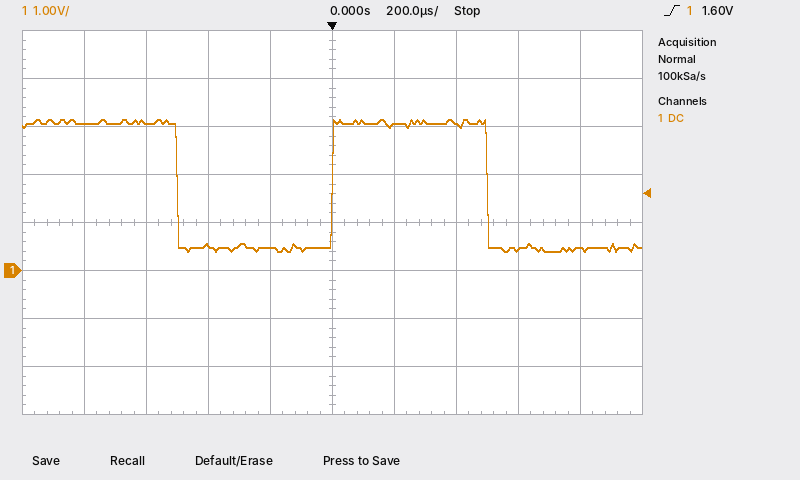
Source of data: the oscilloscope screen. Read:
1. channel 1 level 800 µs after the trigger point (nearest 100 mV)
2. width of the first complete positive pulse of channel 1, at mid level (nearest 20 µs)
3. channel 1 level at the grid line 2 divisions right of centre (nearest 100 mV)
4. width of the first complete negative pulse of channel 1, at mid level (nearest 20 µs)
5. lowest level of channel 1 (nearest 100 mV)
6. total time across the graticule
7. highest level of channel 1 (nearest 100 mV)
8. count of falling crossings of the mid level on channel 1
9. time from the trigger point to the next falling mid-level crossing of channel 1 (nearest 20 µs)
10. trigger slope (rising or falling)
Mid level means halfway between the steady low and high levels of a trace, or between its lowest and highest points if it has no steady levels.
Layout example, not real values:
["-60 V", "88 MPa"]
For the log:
["500 mV", "500 µs", "3.1 V", "500 µs", "400 mV", "2 ms", "3.1 V", "2", "500 µs", "rising"]
